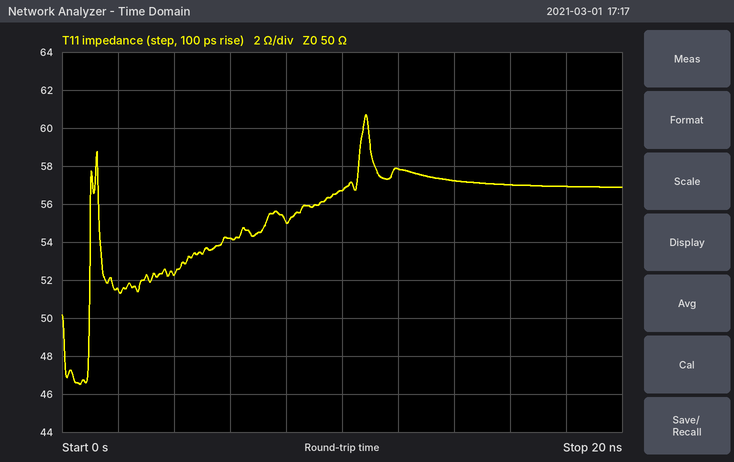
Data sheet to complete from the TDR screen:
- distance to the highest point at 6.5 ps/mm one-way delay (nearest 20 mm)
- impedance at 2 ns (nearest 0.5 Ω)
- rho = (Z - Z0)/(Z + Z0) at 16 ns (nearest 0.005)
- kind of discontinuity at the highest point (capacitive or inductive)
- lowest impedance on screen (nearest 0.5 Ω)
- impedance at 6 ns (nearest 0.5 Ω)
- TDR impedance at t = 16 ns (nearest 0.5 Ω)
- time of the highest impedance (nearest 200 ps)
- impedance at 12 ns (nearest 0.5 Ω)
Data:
840 mm
51.5 Ω
+0.065
inductive
46.5 Ω
54.0 Ω
57.0 Ω
10.8 ns
58.0 Ω
